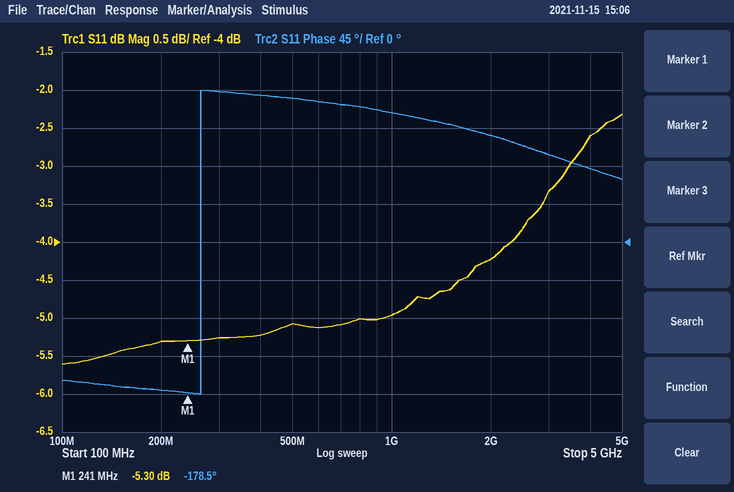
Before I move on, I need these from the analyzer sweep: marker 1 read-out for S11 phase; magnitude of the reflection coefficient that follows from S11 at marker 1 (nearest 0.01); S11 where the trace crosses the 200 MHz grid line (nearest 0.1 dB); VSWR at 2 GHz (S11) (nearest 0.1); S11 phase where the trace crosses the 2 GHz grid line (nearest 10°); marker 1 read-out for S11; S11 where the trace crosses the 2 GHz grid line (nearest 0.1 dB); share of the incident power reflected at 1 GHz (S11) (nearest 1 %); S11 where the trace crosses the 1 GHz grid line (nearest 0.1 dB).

-178.5°
0.54
-5.3 dB
4.2
130°
-5.30 dB
-4.2 dB
32 %
-5.0 dB
